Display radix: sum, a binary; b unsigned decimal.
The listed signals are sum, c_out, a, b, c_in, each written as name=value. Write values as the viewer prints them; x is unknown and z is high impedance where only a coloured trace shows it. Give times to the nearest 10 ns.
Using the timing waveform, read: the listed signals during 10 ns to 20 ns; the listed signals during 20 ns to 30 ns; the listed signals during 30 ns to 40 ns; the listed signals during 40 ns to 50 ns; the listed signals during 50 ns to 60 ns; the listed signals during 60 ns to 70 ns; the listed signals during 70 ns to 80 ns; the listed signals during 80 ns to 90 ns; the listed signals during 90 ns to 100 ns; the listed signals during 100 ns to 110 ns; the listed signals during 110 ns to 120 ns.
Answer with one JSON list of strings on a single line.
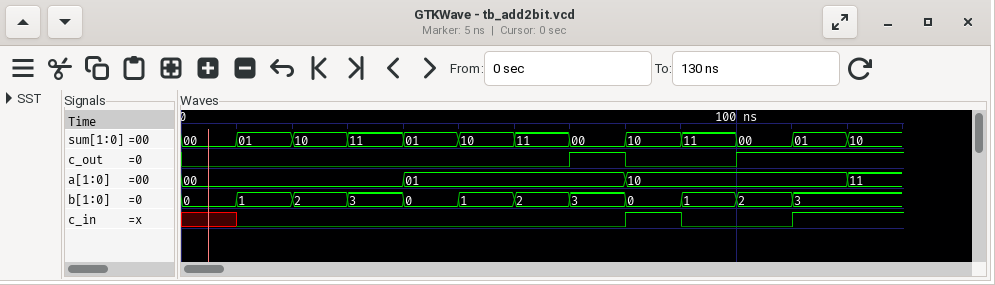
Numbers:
["sum=01, c_out=0, a=00, b=1, c_in=0", "sum=10, c_out=0, a=00, b=2, c_in=0", "sum=11, c_out=0, a=00, b=3, c_in=0", "sum=01, c_out=0, a=01, b=0, c_in=0", "sum=10, c_out=0, a=01, b=1, c_in=0", "sum=11, c_out=0, a=01, b=2, c_in=0", "sum=00, c_out=1, a=01, b=3, c_in=0", "sum=10, c_out=0, a=10, b=0, c_in=1", "sum=11, c_out=0, a=10, b=1, c_in=0", "sum=00, c_out=1, a=10, b=2, c_in=0", "sum=01, c_out=1, a=10, b=3, c_in=1"]
